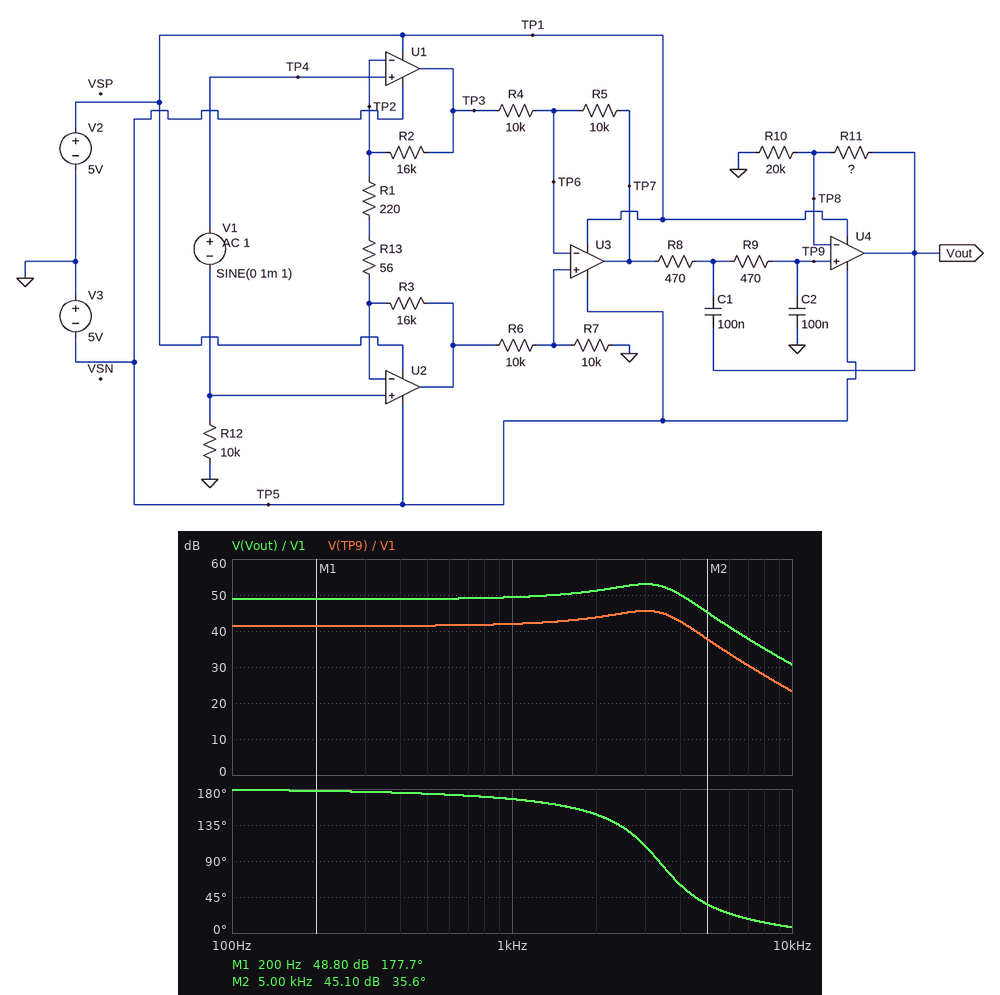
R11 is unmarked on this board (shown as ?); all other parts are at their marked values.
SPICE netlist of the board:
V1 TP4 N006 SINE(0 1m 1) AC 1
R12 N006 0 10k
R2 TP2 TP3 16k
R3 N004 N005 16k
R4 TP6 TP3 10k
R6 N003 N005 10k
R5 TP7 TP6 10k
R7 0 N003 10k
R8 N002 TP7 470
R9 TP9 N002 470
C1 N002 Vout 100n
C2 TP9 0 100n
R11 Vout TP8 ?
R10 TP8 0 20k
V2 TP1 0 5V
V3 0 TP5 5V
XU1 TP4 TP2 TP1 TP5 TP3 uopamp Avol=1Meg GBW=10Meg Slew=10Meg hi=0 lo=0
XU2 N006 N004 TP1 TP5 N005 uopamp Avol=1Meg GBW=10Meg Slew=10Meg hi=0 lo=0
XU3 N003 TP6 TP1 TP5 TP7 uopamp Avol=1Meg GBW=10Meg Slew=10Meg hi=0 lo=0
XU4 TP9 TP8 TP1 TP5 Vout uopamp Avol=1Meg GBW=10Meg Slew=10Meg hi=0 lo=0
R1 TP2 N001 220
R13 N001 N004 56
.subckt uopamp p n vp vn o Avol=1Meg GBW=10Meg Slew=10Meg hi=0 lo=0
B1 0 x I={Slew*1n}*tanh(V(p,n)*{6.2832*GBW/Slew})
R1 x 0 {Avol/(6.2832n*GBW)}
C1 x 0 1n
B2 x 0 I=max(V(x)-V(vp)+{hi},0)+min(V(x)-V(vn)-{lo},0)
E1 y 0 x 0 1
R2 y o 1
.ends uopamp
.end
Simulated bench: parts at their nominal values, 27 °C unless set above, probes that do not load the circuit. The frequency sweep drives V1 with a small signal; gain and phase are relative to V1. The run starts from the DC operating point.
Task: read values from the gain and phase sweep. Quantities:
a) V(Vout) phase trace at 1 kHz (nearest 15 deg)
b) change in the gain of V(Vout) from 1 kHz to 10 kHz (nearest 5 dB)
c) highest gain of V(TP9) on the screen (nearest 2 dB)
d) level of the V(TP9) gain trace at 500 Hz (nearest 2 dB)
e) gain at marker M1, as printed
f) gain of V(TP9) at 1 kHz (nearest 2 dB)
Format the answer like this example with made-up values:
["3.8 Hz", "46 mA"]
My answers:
["165 deg", "-20 dB", "46 dB", "42 dB", "48.80 dB", "42 dB"]
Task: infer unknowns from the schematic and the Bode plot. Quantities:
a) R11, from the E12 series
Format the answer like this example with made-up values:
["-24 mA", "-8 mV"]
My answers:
["27 kΩ"]
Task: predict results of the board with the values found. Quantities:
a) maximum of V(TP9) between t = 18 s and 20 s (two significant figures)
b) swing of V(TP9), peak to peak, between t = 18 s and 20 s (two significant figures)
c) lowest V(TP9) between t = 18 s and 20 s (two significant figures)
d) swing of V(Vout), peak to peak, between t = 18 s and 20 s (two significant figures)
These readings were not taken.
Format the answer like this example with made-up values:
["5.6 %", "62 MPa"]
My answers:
["120 mV", "230 mV", "-120 mV", "550 mV"]
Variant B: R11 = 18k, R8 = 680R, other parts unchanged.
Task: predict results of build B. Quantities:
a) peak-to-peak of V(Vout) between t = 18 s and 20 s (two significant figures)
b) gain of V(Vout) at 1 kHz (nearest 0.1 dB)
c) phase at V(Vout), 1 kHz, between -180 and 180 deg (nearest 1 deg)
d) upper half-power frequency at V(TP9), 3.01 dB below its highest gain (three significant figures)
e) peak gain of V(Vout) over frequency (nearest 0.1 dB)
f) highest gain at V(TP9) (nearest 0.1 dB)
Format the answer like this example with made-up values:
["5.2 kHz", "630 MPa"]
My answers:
["440 mV", "47.5 dB", "158 deg", "3.31 kHz", "48.5 dB", "42.9 dB"]
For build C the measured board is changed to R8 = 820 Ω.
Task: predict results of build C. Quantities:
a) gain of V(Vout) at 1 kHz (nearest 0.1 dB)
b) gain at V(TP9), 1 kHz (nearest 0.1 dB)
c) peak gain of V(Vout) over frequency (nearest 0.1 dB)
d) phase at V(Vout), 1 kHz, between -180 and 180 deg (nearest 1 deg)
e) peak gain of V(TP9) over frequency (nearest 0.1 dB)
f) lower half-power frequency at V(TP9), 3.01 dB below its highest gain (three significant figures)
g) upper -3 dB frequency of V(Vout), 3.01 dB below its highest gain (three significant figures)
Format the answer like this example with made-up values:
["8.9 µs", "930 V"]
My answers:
["50.1 dB", "42.7 dB", "59.5 dB", "172 deg", "52.1 dB", "2.09 kHz", "2.86 kHz"]
